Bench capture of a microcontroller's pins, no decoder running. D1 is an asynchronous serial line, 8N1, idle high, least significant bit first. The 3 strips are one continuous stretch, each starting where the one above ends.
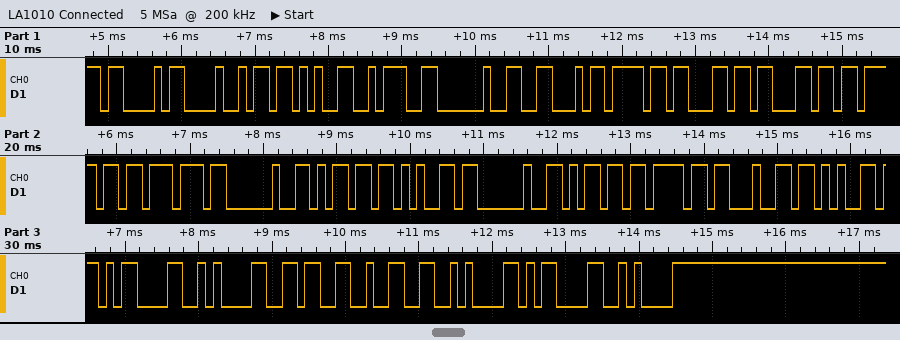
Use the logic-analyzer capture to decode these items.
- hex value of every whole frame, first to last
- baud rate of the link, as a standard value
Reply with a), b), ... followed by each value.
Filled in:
a) 43 48 2B 3A 20 46 6F 6C 6C 6F 77 20 6D 65 20 6D 6F 64 65 0D 0A 36 32 0A 0D 0A
b) 9600 baud
